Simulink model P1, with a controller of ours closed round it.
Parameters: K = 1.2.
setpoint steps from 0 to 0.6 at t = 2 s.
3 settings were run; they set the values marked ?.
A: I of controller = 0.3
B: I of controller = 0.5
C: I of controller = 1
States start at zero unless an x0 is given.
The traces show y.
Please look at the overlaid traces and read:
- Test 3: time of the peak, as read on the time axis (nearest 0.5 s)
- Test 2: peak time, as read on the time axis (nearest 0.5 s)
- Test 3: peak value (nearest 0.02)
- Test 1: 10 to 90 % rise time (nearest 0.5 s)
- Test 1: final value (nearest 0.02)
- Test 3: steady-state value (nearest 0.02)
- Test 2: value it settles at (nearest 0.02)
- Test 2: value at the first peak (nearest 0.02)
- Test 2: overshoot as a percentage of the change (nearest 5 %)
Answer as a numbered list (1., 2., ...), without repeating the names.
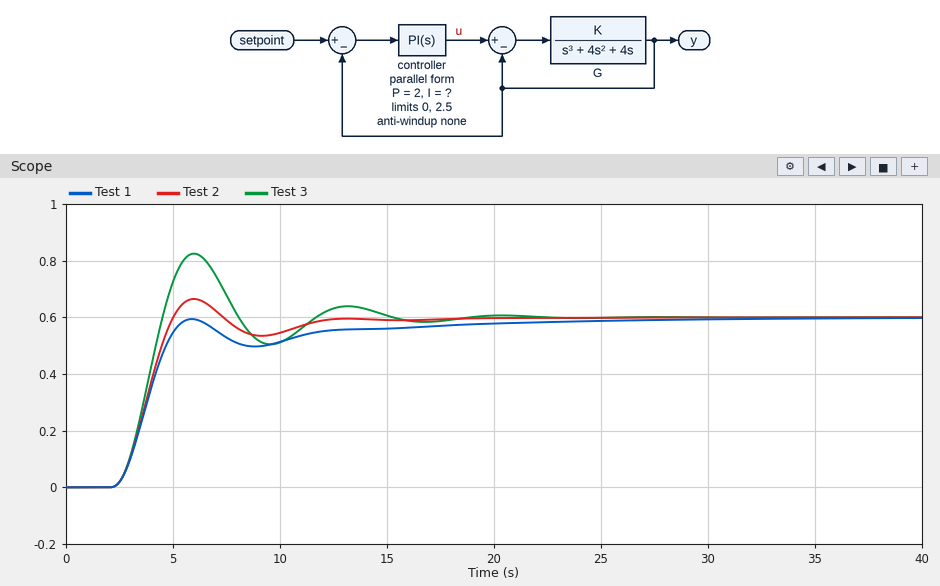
1. 6.0 s
2. 6.0 s
3. 0.82
4. 2.0 s
5. 0.60
6. 0.60
7. 0.60
8. 0.66
9. 10 %
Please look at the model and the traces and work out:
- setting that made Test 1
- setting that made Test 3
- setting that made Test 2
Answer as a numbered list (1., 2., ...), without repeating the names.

1. A
2. C
3. B
